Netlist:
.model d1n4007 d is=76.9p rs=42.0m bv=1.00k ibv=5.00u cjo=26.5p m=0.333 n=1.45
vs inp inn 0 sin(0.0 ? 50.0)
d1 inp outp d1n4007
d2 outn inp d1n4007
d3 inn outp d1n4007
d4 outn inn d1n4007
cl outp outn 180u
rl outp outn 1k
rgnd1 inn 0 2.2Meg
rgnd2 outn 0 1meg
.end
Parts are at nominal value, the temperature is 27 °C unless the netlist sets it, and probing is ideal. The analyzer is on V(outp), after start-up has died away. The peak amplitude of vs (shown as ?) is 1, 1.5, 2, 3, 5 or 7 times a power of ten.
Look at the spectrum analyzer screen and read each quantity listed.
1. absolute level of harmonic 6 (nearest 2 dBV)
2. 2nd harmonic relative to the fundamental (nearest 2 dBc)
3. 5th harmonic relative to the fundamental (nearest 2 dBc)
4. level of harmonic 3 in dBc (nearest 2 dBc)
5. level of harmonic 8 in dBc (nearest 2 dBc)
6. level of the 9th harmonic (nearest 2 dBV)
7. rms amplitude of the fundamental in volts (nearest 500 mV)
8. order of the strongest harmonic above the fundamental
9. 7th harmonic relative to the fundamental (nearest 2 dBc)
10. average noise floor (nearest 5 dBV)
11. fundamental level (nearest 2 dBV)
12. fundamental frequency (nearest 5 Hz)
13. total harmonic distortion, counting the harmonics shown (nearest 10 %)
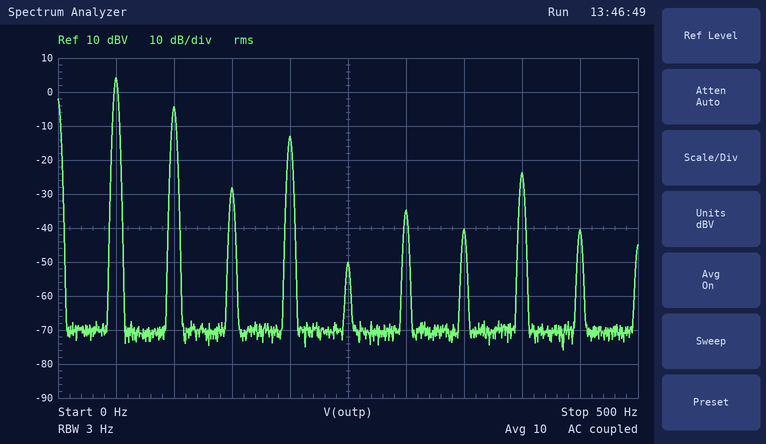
-34 dBV
-8 dBc
-54 dBc
-32 dBc
-28 dBc
-40 dBV
1.5 V
2
-44 dBc
-70 dBV
4 dBV
50 Hz
40 %
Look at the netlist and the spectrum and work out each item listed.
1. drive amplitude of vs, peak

15 V
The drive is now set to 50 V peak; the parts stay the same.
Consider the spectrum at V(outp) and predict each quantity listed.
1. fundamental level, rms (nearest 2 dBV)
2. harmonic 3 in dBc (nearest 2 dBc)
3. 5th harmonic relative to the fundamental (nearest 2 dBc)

14 dBV
-40 dBc
-56 dBc
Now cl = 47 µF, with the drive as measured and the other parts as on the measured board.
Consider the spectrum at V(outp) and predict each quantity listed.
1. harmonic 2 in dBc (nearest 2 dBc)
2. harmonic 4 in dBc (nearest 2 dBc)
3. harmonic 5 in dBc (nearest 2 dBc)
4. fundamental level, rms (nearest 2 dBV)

-10 dBc
-12 dBc
-50 dBc
4 dBV
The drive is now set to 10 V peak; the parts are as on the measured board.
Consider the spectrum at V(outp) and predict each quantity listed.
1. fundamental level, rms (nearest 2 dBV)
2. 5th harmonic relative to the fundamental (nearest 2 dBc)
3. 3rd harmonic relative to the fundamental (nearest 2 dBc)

0 dBV
-46 dBc
-30 dBc
